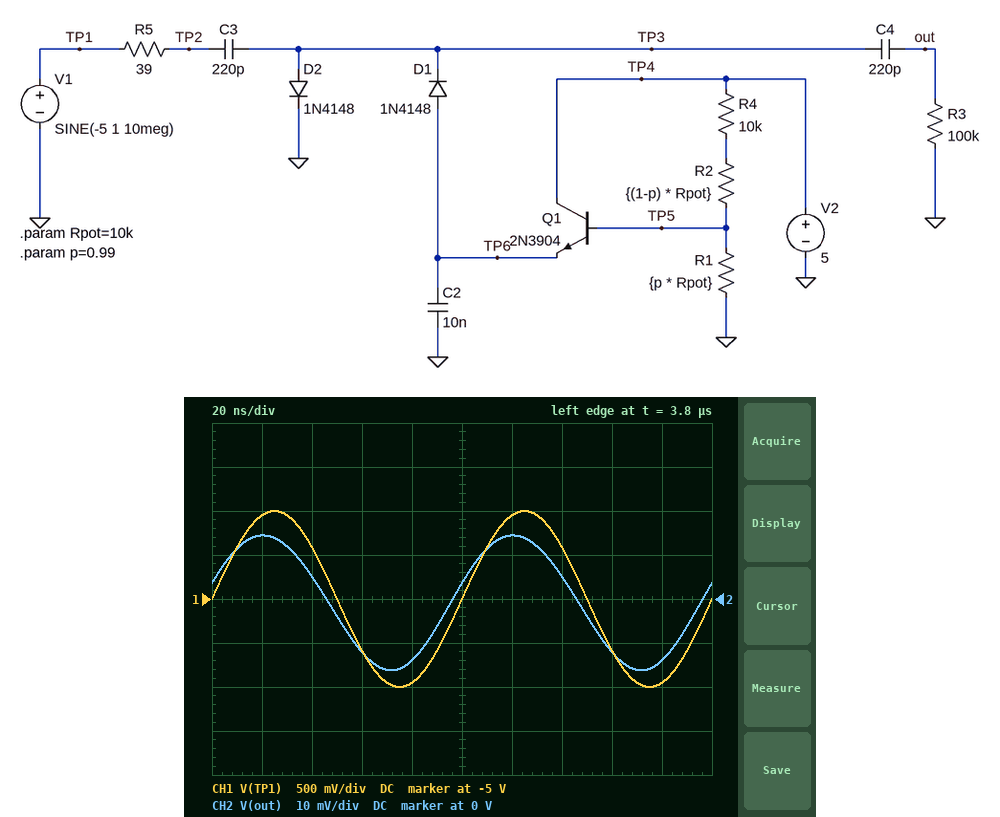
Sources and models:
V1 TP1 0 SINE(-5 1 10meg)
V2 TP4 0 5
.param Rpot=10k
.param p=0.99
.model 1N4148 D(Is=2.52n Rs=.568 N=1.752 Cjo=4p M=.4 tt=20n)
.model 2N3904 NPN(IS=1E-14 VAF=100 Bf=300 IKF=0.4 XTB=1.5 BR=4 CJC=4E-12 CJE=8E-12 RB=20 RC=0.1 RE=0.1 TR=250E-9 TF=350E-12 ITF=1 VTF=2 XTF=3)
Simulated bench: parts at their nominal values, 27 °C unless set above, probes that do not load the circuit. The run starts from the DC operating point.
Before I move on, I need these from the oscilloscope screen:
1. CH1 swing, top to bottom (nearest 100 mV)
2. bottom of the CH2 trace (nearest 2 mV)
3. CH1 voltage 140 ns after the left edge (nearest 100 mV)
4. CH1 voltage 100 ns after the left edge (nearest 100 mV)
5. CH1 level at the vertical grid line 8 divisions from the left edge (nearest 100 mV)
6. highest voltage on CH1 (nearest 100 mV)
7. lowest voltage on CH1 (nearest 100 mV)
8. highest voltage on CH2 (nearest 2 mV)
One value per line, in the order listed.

2.0 V
-16 mV
-4.4 V
-5.0 V
-5.6 V
-4.0 V
-6.0 V
14 mV
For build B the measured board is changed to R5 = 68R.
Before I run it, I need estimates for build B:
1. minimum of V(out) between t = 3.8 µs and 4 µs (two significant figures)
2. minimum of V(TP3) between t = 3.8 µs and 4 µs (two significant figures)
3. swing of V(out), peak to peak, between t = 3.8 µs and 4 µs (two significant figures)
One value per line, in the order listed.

-13 mV
710 mV
25 mV
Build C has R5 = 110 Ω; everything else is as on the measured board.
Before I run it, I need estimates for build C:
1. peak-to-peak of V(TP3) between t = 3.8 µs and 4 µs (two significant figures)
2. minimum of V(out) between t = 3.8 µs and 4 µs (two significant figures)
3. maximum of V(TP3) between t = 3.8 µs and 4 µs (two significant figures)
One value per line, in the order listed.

19 mV
-9.9 mV
730 mV
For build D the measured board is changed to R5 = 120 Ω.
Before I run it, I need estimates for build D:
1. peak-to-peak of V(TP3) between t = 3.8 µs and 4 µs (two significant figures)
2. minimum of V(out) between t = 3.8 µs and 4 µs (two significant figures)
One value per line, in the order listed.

18 mV
-9.3 mV
